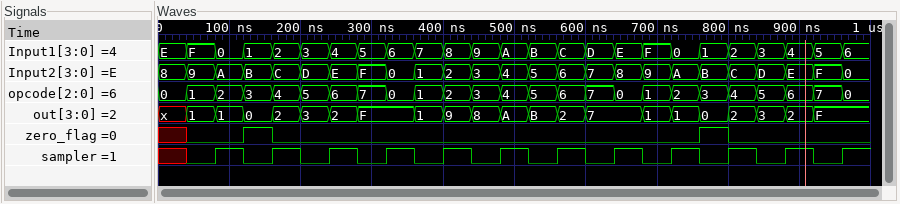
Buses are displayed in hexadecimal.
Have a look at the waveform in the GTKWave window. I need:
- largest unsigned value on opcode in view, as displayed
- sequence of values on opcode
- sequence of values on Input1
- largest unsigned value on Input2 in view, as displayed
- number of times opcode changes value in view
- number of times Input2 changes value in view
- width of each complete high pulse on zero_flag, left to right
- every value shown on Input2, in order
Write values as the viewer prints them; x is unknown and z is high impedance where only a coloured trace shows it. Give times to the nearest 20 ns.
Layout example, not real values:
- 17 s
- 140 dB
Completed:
- 7
- 0, 1, 2, 3, 4, 5, 6, 7, 0, 1, 2, 3, 4, 5, 6, 7, 0, 1, 2, 3, 4, 5, 6, 7, 0
- E, F, 0, 1, 2, 3, 4, 5, 6, 7, 8, 9, A, B, C, D, E, F, 0, 1, 2, 3, 4, 5, 6
- F
- 24
- 24
- 40 ns, 40 ns
- 8, 9, A, B, C, D, E, F, 0, 1, 2, 3, 4, 5, 6, 7, 8, 9, A, B, C, D, E, F, 0
